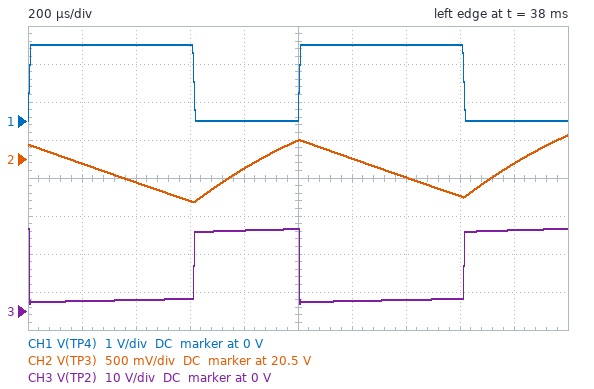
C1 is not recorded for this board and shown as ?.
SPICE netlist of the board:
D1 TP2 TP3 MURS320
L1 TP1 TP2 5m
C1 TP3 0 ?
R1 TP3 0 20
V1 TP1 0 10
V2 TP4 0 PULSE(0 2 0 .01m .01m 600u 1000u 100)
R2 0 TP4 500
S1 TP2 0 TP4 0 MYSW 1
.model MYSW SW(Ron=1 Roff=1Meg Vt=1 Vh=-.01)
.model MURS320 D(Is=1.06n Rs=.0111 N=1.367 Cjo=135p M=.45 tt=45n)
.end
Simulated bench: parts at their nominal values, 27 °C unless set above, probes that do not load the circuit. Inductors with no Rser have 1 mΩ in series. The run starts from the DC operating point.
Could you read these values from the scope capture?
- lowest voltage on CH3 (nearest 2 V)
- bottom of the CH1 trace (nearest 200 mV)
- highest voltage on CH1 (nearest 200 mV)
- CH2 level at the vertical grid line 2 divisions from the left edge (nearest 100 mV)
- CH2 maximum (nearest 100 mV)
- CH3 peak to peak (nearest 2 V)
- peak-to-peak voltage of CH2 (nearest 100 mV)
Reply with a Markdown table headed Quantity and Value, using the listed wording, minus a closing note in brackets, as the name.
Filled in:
| Quantity | Value |
|---|---|
| lowest voltage on CH3 | 2 V |
| bottom of the CH1 trace | 0 V |
| highest voltage on CH1 | 2.0 V |
| CH2 level at the vertical grid line 2 divisions from the left edge | 20.2 V |
| CH2 maximum | 20.8 V |
| CH3 peak to peak | 20 V |
| peak-to-peak voltage of CH2 | 900 mV |
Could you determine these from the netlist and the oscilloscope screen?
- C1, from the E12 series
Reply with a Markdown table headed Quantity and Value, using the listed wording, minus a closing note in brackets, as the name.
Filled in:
| Quantity | Value |
|---|---|
| C1, from the E12 series | 820 µF |
